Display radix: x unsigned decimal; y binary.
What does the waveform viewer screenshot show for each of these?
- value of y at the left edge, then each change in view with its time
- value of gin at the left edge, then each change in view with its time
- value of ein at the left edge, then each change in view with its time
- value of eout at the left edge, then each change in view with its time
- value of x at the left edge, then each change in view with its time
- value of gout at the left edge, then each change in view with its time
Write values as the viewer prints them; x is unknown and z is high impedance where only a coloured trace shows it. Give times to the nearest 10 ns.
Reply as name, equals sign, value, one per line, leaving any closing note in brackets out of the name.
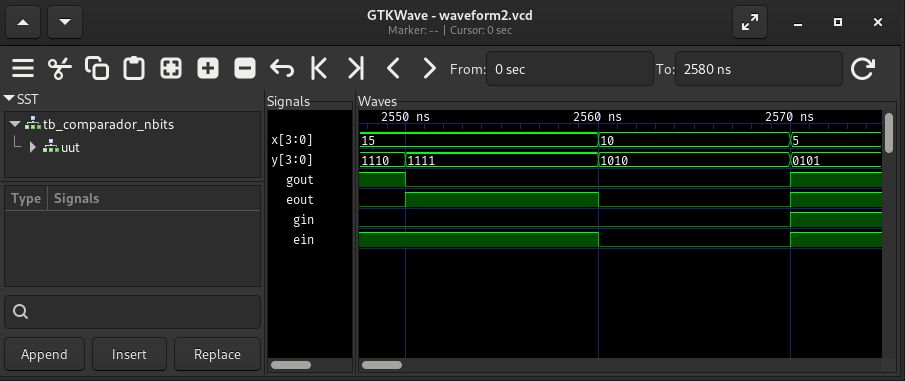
value of y at the left edge, then each change in view with its time = 1110, 1111 at 2550 ns, 1010 at 2560 ns, 0101 at 2570 ns
value of gin at the left edge, then each change in view with its time = 0, 1 at 2570 ns
value of ein at the left edge, then each change in view with its time = 1, 0 at 2560 ns, 1 at 2570 ns
value of eout at the left edge, then each change in view with its time = 0, 1 at 2550 ns, 0 at 2560 ns, 1 at 2570 ns
value of x at the left edge, then each change in view with its time = 15, 10 at 2560 ns, 5 at 2570 ns
value of gout at the left edge, then each change in view with its time = 1, 0 at 2550 ns, 1 at 2570 ns
